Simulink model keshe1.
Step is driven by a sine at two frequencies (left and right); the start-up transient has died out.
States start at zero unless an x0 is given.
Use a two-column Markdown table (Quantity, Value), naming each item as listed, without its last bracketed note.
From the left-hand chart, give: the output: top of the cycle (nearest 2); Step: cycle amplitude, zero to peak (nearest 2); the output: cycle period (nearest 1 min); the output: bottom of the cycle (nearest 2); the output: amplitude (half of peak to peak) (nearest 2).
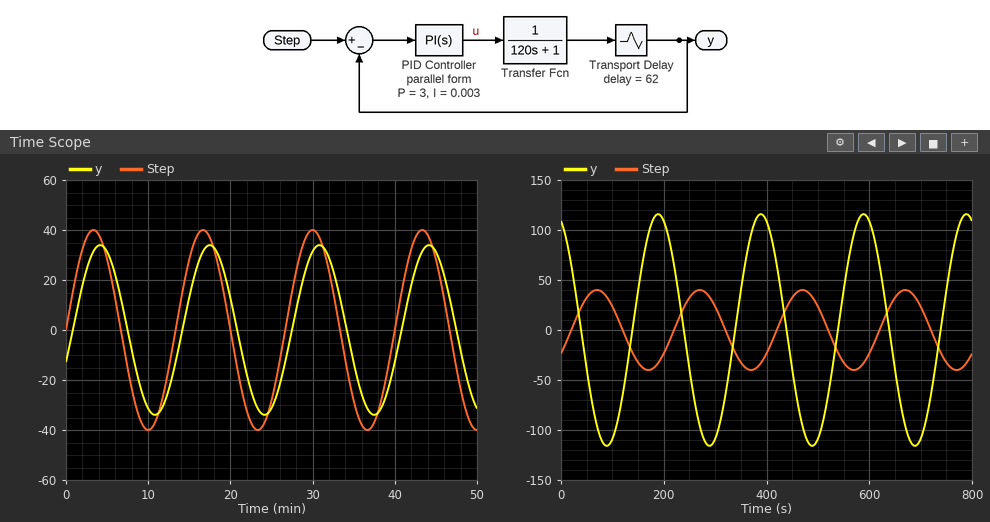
| Quantity | Value |
|---|---|
| the output: top of the cycle | 34 |
| Step: cycle amplitude, zero to peak | 40 |
| the output: cycle period | 13 min |
| the output: bottom of the cycle | -34 |
| the output: amplitude (half of peak to peak) | 34 |
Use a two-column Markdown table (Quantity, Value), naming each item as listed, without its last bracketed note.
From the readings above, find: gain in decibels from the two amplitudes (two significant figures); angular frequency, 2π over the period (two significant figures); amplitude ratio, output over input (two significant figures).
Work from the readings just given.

| Quantity | Value |
|---|---|
| gain in decibels from the two amplitudes | -1.4 dB |
| angular frequency, 2π over the period | 0.48 rad/min |
| amplitude ratio, output over input | 0.85 |
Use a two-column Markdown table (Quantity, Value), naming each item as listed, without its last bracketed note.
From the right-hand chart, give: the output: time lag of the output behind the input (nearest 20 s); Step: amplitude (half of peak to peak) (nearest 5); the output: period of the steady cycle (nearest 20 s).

| Quantity | Value |
|---|---|
| the output: time lag of the output behind the input | 120 s |
| Step: amplitude (half of peak to peak) | 40 |
| the output: period of the steady cycle | 200 s |
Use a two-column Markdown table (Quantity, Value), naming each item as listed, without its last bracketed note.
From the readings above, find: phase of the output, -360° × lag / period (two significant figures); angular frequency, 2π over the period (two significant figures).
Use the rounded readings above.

| Quantity | Value |
|---|---|
| phase of the output, -360° × lag / period | -220° |
| angular frequency, 2π over the period | 0.031 rad/s |
